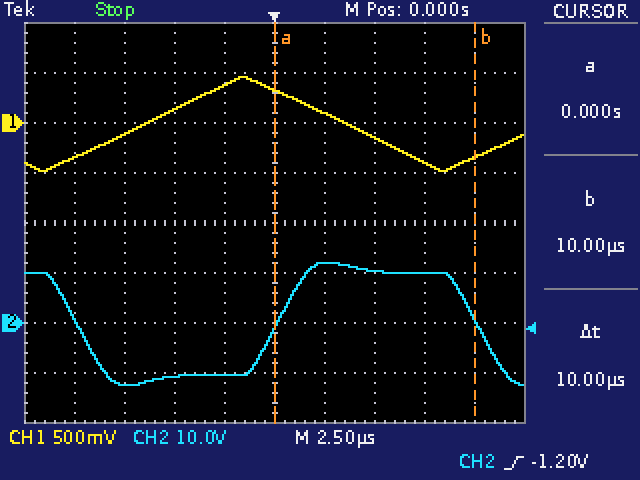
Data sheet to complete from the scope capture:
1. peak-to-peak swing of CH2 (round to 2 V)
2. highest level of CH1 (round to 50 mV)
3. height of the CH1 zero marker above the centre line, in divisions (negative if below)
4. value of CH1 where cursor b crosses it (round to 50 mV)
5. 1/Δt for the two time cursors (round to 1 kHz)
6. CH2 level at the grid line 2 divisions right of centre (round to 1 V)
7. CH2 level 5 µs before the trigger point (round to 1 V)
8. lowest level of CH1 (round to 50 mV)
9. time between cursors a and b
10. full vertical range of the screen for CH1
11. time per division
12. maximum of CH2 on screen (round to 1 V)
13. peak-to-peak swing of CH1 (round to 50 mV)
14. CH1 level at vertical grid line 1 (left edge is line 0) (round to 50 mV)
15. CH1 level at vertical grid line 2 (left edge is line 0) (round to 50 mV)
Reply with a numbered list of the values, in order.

1. 24 V
2. 450 mV
3. +2.0 div
4. -350 mV
5. 100 kHz
6. 10 V
7. -11 V
8. -500 mV
9. 10 µs
10. 4 V
11. 2.5 µs
12. 12 V
13. 950 mV
14. -350 mV
15. -100 mV
